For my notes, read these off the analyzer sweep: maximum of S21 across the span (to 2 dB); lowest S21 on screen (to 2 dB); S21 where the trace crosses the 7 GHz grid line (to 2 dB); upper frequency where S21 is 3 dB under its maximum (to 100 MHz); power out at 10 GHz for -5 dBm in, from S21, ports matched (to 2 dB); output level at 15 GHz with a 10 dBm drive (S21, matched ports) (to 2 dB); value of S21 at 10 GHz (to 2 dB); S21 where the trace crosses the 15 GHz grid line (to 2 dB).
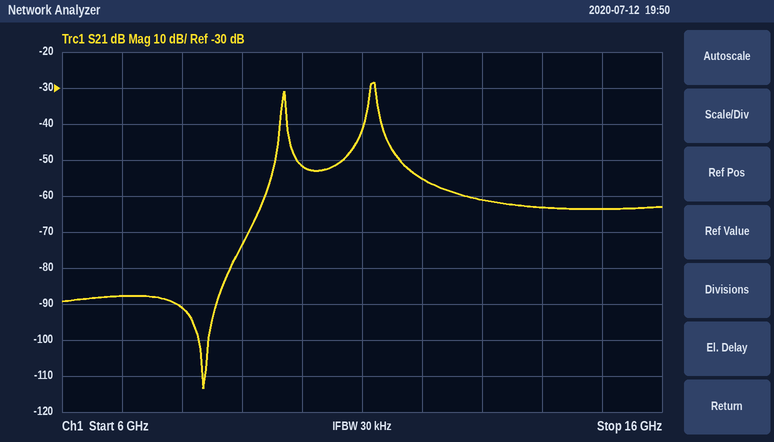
-28 dB
-114 dB
-88 dB
11.2 GHz
-56 dBm
-54 dBm
-52 dB
-64 dB
